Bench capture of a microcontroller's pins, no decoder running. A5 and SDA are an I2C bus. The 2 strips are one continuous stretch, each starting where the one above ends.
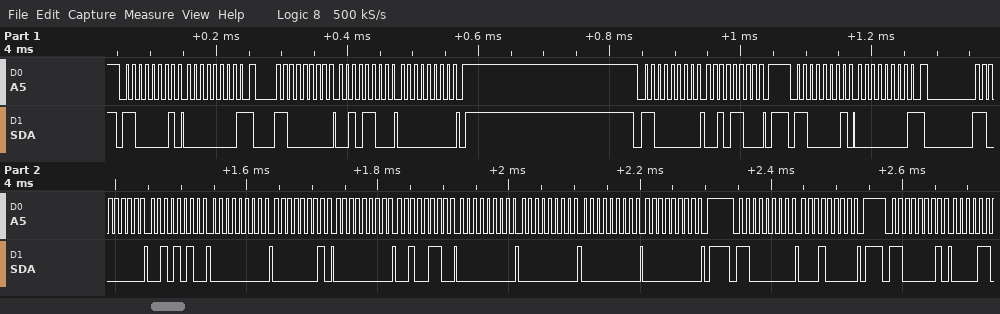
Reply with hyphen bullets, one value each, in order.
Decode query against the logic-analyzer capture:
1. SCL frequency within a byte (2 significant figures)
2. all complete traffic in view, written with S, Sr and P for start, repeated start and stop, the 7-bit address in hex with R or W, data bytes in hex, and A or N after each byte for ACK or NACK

- 100 kHz
- S 60R A 00 N Sr 60W A 2C A 00 A P S 60W A 2C A P S 60R A 00 N Sr 60W A 2A A 00 A 01 A 00 A 26 A 00 A 00 A 00 A 00 A P S 60W A 10 A P S 60R A
